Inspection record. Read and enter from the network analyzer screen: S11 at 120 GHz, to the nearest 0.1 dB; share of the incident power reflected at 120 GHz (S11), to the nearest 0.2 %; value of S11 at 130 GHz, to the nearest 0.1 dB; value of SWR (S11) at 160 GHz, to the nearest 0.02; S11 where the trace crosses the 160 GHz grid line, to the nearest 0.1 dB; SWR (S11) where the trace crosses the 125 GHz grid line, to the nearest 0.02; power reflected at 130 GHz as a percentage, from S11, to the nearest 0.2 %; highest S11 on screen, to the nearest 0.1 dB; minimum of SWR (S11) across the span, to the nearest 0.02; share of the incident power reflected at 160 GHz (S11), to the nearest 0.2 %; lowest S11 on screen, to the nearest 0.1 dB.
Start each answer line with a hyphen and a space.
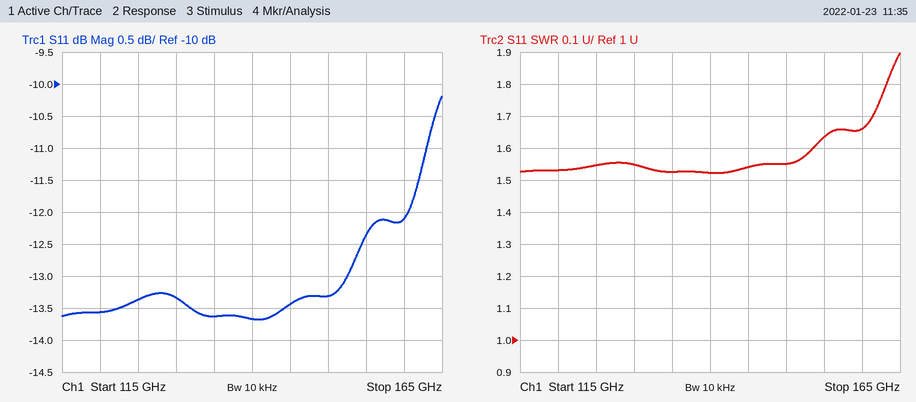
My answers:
- -13.6 dB
- 4.4 %
- -13.3 dB
- 1.66
- -12.1 dB
- 1.54
- 4.6 %
- -10.2 dB
- 1.52
- 6.2 %
- -13.7 dB
